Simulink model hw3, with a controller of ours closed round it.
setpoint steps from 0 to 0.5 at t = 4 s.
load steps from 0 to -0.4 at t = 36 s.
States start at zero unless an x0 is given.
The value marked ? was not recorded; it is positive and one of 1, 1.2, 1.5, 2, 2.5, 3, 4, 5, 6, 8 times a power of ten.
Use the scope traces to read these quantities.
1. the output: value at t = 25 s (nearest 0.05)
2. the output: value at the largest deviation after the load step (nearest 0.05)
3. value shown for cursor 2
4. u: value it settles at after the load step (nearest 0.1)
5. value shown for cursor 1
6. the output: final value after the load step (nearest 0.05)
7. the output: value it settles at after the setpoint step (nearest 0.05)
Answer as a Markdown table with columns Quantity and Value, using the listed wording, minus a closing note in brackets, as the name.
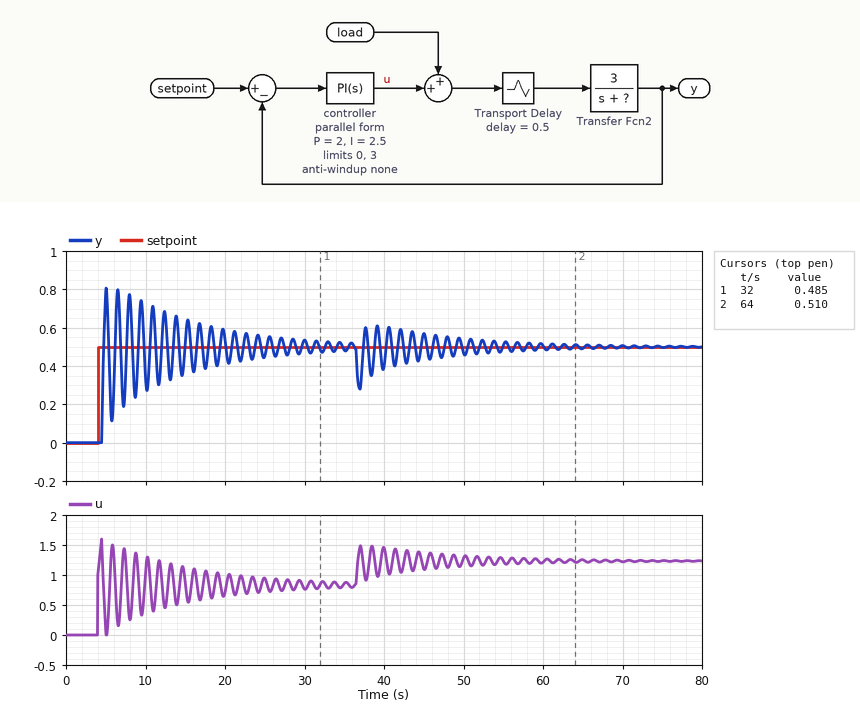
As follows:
| Quantity | Value |
|---|---|
| the output: value at t = 25 s | 0.45 |
| the output: value at the largest deviation after the load step | 0.30 |
| value shown for cursor 2 | 0.510 |
| u: value it settles at after the load step | 1.2 |
| value shown for cursor 1 | 0.485 |
| the output: final value after the load step | 0.50 |
| the output: value it settles at after the setpoint step | 0.50 |
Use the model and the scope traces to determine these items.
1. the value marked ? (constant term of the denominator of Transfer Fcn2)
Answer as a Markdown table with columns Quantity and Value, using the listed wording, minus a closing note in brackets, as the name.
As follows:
| Quantity | Value |
|---|---|
| the value marked ? | 5 |
